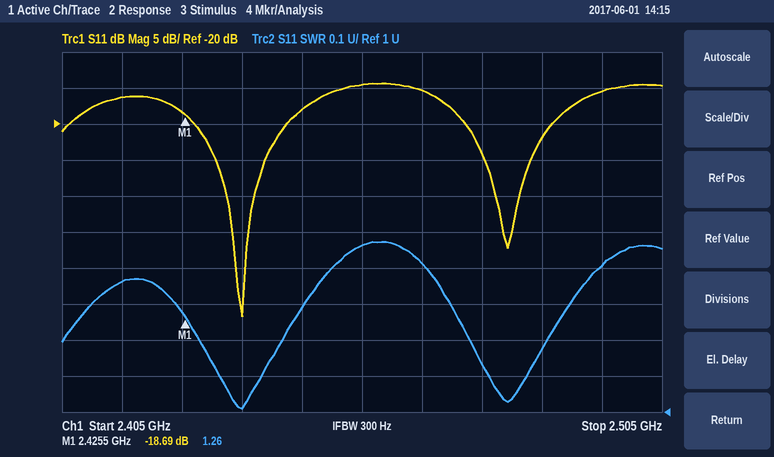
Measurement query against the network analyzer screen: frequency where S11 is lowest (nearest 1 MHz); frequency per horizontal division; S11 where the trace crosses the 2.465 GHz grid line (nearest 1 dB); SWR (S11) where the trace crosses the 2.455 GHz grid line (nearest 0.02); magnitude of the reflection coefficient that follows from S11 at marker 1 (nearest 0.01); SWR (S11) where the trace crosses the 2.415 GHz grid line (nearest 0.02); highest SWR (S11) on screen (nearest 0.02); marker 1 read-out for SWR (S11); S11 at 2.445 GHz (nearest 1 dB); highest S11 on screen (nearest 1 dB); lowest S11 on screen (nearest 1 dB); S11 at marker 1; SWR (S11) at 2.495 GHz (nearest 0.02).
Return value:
2.435 GHz
10 MHz
-15 dB
1.46
0.12
1.36
1.48
1.26
-18 dB
-14 dB
-47 dB
-18.69 dB
1.40
